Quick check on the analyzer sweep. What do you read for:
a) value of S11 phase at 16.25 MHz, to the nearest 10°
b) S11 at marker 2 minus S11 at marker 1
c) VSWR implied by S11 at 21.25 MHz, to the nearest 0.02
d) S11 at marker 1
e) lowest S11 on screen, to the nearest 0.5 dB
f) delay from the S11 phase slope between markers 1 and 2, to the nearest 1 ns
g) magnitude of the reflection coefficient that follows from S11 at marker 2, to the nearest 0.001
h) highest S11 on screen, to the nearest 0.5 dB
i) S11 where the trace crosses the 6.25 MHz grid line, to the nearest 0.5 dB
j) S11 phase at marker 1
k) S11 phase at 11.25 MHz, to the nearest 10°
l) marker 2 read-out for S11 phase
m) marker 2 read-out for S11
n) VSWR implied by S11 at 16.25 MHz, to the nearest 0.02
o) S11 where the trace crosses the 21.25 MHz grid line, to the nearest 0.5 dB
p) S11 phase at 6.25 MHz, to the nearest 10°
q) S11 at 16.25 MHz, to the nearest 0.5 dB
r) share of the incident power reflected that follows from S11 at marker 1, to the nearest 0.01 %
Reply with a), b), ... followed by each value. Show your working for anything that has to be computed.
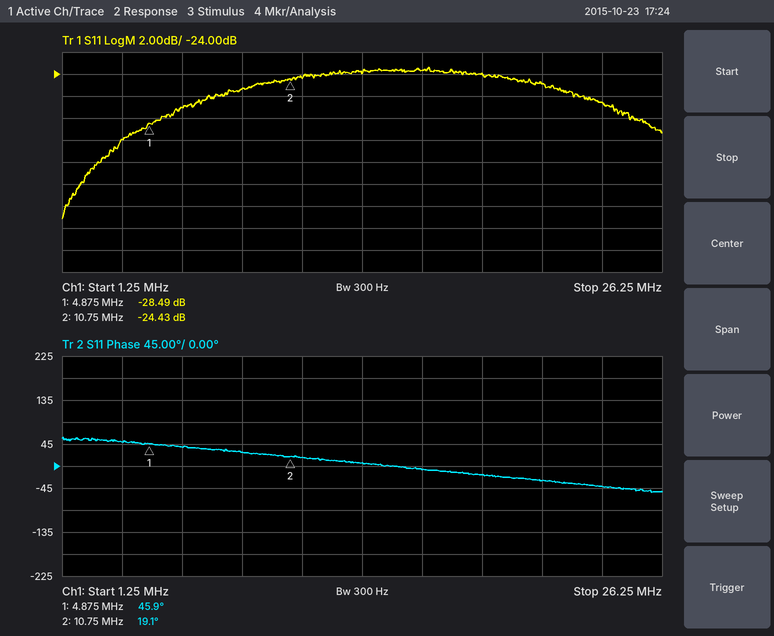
a) -10°
b) -24.43 − (-28.49) = 4.06 dB
c) |Γ| = 10^(-25/20) = 0.0562; VSWR = (1 + 0.0562)/(1 − 0.0562) ≈ 1.12
d) -28.49 dB
e) -37.0 dB
f) −(19.1° − (45.9°))/(360° × 5.875 MHz) ≈ 13 ns
g) 10^(-24.43/20) ≈ 0.060
h) -23.5 dB
i) -27.0 dB
j) 45.9°
k) 20°
l) 19.1°
m) -24.43 dB
n) |Γ| = 10^(-23.5/20) = 0.0668; VSWR = (1 + 0.0668)/(1 − 0.0668) ≈ 1.14
o) -25.0 dB
p) 40°
q) -23.5 dB
r) 10^(-28.49/10) ≈ 0.14 %
